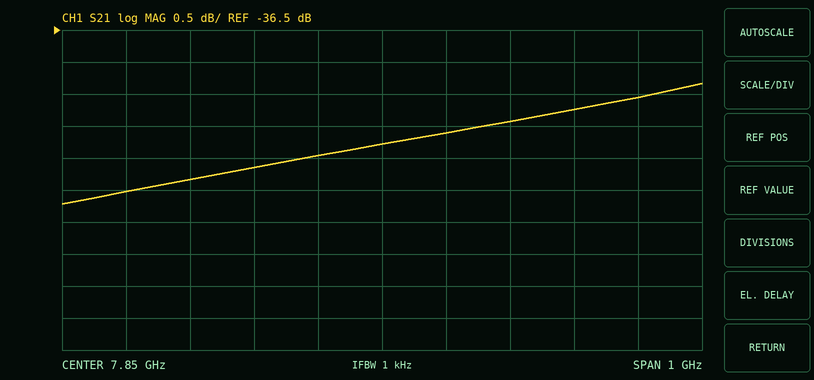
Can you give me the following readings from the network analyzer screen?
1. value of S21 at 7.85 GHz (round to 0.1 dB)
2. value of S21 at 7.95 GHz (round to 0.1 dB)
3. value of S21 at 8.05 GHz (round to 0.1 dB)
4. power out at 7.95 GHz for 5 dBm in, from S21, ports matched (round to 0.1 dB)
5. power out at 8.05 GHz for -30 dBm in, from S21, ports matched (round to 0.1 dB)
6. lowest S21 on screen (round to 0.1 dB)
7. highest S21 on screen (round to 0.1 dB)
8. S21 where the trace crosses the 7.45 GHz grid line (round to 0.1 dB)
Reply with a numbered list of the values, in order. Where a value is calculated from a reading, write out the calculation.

1. -38.3 dB
2. -38.1 dB
3. -37.9 dB
4. 5 dBm + (-38.1 dB) = -33.1 dBm
5. -30 dBm + (-37.9 dB) = -67.9 dBm
6. -39.2 dB
7. -37.3 dB
8. -39.0 dB
